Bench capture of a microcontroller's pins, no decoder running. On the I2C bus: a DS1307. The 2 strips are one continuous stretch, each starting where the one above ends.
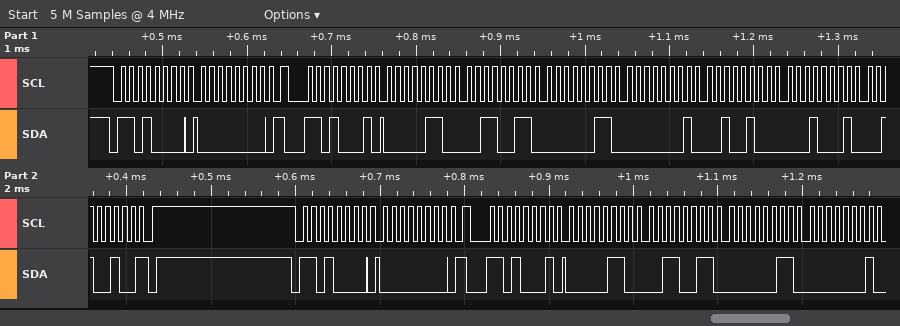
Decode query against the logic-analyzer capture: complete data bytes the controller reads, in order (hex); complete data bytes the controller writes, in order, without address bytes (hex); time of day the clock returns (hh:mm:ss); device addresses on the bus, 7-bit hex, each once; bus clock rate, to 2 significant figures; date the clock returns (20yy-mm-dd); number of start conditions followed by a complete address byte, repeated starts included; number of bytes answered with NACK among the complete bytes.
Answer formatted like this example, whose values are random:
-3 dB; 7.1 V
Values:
06 33 03 01 24 11 24 06 33 03 01; 00 00; 03:33:06; 0x68; 100 kHz; 2024-11-24; 4; 1
